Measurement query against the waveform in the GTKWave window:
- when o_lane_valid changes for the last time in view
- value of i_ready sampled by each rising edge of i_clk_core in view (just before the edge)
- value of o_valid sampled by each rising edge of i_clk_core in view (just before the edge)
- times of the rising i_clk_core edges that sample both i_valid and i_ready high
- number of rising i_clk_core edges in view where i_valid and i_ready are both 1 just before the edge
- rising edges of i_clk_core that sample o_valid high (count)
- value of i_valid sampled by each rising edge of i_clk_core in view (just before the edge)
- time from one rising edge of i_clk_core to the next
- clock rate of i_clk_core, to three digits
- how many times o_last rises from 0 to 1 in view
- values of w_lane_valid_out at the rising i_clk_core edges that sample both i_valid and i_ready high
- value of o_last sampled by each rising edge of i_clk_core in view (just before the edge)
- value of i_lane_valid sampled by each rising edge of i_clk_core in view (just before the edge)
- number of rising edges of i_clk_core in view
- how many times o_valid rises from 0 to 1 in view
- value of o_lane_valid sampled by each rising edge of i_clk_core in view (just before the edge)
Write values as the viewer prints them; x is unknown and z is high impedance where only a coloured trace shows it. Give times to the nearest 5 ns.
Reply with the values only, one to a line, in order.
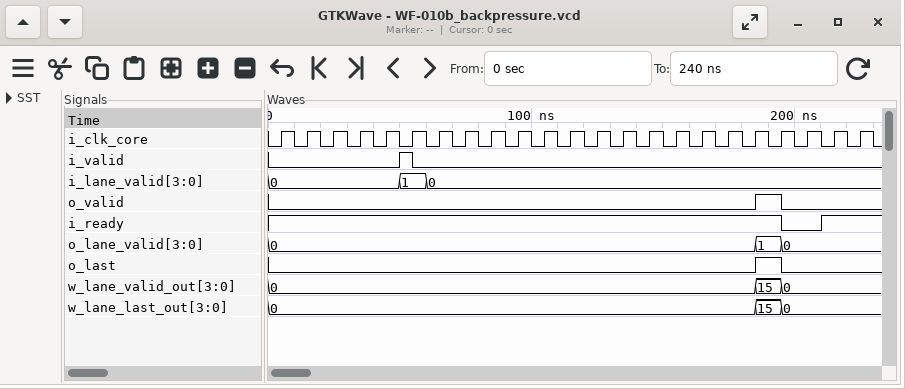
195 ns
1 1 1 1 1 1 1 1 1 1 1 1 1 1 1 1 1 1 1 1 0 1 1
0 0 0 0 0 0 0 0 0 0 0 0 0 0 0 0 0 0 0 1 0 0 0
55 ns
1
1
0 0 0 0 0 1 0 0 0 0 0 0 0 0 0 0 0 0 0 0 0 0 0
10 ns
100 MHz
1
0
0 0 0 0 0 0 0 0 0 0 0 0 0 0 0 0 0 0 0 1 0 0 0
0, 0, 0, 0, 0, 1, 0, 0, 0, 0, 0, 0, 0, 0, 0, 0, 0, 0, 0, 0, 0, 0, 0
23
1
0, 0, 0, 0, 0, 0, 0, 0, 0, 0, 0, 0, 0, 0, 0, 0, 0, 0, 0, 1, 0, 0, 0
